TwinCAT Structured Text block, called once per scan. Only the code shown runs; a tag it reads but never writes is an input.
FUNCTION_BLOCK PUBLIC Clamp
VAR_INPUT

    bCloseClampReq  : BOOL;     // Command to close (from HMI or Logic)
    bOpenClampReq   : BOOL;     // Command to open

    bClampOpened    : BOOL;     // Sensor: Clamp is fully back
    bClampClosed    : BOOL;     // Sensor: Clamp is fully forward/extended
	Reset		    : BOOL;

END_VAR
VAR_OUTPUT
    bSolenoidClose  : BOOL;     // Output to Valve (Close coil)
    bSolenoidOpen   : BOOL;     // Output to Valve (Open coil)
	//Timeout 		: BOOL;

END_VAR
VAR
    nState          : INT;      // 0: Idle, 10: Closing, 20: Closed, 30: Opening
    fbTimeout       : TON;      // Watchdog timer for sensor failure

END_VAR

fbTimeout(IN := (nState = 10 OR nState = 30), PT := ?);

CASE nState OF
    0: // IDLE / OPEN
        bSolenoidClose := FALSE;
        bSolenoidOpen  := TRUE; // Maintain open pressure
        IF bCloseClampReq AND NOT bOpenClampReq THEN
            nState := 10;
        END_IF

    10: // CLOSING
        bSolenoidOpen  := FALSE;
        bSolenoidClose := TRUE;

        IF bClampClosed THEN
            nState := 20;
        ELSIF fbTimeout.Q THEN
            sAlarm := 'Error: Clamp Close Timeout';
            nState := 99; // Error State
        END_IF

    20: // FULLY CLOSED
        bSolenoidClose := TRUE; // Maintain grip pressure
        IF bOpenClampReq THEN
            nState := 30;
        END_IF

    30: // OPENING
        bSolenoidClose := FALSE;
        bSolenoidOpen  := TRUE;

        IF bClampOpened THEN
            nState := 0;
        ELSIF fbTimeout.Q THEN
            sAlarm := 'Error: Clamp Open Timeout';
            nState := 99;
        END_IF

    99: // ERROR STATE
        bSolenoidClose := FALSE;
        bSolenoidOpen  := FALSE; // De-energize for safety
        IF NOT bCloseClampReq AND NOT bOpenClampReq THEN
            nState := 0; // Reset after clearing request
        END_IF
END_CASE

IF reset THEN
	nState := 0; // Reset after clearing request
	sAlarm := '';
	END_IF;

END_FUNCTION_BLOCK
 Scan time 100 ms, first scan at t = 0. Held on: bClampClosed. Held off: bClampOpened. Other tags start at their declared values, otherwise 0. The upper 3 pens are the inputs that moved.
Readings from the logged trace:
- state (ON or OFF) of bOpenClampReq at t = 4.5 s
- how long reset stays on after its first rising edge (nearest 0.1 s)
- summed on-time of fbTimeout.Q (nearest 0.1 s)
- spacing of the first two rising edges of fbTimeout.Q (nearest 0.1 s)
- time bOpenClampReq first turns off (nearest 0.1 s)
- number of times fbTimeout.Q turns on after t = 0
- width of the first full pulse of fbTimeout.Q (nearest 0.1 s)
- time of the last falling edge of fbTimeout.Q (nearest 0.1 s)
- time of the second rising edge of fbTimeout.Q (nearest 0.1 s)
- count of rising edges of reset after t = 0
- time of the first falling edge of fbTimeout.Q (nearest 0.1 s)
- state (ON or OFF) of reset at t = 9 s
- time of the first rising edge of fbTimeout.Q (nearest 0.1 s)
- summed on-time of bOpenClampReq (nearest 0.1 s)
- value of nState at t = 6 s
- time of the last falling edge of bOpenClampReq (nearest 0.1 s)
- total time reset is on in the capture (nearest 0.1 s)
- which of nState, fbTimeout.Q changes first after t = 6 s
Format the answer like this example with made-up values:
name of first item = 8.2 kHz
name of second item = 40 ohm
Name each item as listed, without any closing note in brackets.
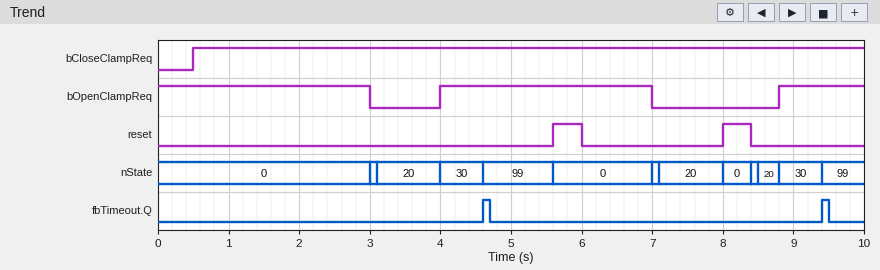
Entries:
state (ON or OFF) of bOpenClampReq at t = 4.5 s = ON
how long reset stays on after its first rising edge = 0.4 s
summed on-time of fbTimeout.Q = 0.2 s
spacing of the first two rising edges of fbTimeout.Q = 4.8 s
time bOpenClampReq first turns off = 3.0 s
number of times fbTimeout.Q turns on after t = 0 = 2
width of the first full pulse of fbTimeout.Q = 0.1 s
time of the last falling edge of fbTimeout.Q = 9.5 s
time of the second rising edge of fbTimeout.Q = 9.4 s
count of rising edges of reset after t = 0 = 2
time of the first falling edge of fbTimeout.Q = 4.7 s
state (ON or OFF) of reset at t = 9 s = OFF
time of the first rising edge of fbTimeout.Q = 4.6 s
summed on-time of bOpenClampReq = 7.2 s
value of nState at t = 6 s = 0
time of the last falling edge of bOpenClampReq = 7.0 s
total time reset is on in the capture = 0.8 s
which of nState, fbTimeout.Q changes first after t = 6 s = nState
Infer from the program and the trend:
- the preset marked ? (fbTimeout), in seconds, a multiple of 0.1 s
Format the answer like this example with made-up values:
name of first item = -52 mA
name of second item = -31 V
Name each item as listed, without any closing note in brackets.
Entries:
the preset marked ? (fbTimeout), in seconds, a multiple of 0.1 s = 0.5 s
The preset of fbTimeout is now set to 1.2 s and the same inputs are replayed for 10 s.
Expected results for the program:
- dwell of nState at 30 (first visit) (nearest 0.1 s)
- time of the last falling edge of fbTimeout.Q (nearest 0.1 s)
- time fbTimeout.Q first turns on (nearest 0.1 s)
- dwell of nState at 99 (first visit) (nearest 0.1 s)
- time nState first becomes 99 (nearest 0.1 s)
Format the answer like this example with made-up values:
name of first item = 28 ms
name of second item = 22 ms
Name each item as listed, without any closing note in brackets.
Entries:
dwell of nState at 30 (first visit) = 1.3 s
time of the last falling edge of fbTimeout.Q = 5.4 s
time fbTimeout.Q first turns on = 5.3 s
dwell of nState at 99 (first visit) = 0.3 s
time nState first becomes 99 = 5.3 s
